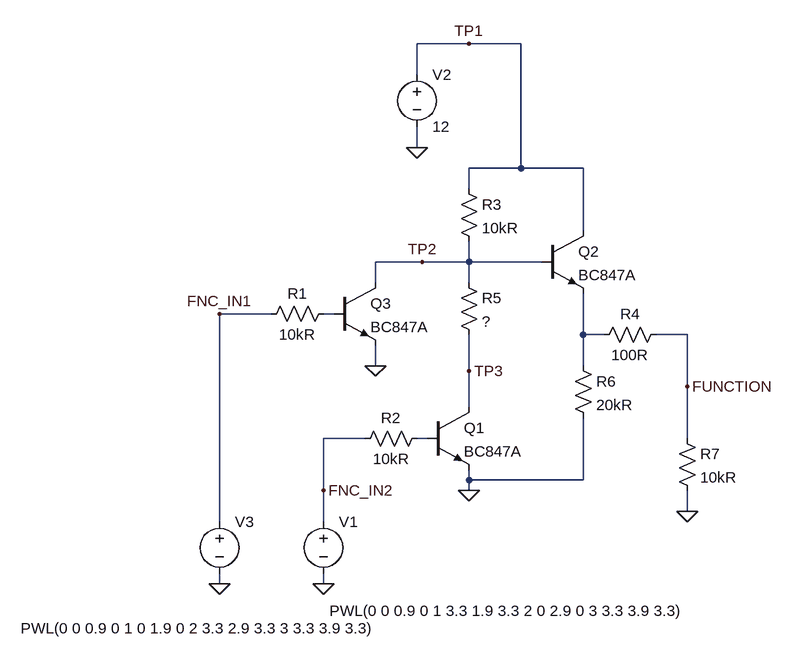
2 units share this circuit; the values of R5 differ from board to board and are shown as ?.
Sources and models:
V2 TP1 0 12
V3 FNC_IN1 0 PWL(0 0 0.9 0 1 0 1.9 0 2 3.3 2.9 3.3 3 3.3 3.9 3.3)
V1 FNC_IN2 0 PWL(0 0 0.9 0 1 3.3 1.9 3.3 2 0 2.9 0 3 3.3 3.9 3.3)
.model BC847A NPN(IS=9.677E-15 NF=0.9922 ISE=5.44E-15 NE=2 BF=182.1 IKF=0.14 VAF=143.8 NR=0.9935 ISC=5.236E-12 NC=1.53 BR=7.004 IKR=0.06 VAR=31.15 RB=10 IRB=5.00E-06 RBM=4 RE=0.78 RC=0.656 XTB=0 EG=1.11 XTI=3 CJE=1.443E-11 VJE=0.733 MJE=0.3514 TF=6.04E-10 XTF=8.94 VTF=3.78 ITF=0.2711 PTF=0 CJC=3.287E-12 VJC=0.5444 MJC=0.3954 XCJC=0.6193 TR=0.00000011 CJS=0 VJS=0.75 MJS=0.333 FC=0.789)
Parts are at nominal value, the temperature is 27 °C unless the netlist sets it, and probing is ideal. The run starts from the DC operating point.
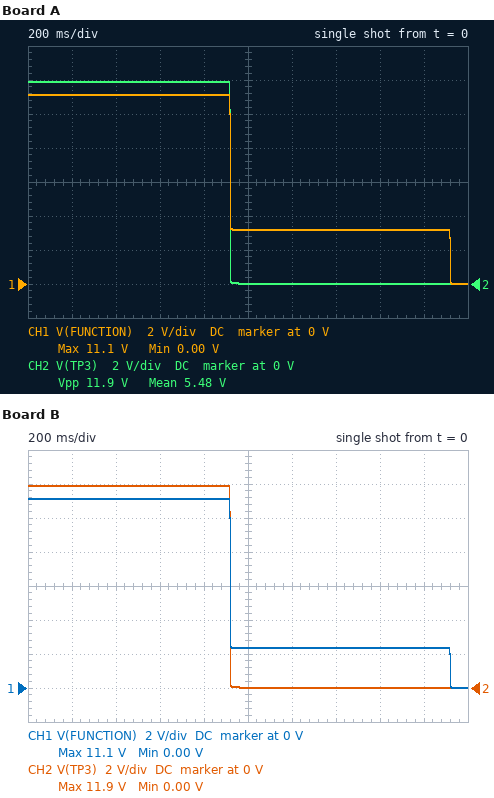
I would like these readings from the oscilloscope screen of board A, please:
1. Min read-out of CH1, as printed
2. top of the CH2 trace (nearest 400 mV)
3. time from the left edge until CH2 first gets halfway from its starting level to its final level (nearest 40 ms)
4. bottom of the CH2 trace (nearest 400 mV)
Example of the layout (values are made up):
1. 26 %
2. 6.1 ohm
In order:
1. 0.00 V
2. 12.0 V
3. 920 ms
4. 0 V
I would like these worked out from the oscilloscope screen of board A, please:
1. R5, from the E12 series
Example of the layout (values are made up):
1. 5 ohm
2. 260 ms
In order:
1. 4.7 kΩ
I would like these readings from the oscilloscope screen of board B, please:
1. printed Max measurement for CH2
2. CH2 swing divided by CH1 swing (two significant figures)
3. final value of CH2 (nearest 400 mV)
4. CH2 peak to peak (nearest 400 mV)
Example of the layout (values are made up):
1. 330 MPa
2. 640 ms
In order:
1. 11.9 V
2. 1.1
3. 0 V
4. 12.0 V
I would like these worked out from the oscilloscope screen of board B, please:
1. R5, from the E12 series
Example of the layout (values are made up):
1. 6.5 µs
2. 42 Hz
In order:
1. 3.3 kΩ
